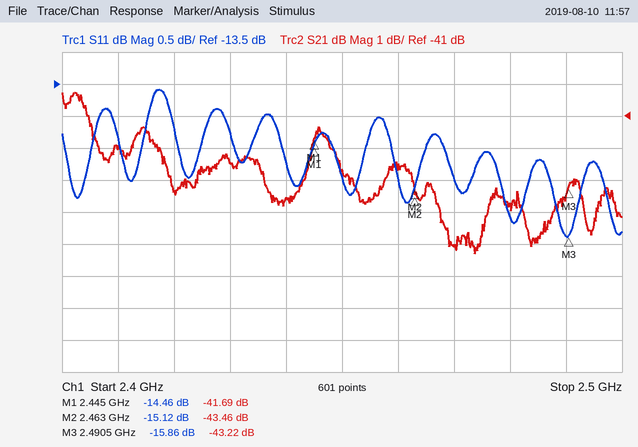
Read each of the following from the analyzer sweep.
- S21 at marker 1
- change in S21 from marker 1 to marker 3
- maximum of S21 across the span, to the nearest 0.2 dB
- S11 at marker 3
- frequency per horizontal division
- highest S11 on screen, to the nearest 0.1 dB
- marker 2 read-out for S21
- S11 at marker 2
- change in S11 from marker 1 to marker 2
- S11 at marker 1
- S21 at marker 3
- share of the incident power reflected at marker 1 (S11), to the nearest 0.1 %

-41.69 dB
-1.53 dB
-40.2 dB
-15.86 dB
10 MHz
-13.6 dB
-43.46 dB
-15.12 dB
-0.66 dB
-14.46 dB
-43.22 dB
3.6 %
